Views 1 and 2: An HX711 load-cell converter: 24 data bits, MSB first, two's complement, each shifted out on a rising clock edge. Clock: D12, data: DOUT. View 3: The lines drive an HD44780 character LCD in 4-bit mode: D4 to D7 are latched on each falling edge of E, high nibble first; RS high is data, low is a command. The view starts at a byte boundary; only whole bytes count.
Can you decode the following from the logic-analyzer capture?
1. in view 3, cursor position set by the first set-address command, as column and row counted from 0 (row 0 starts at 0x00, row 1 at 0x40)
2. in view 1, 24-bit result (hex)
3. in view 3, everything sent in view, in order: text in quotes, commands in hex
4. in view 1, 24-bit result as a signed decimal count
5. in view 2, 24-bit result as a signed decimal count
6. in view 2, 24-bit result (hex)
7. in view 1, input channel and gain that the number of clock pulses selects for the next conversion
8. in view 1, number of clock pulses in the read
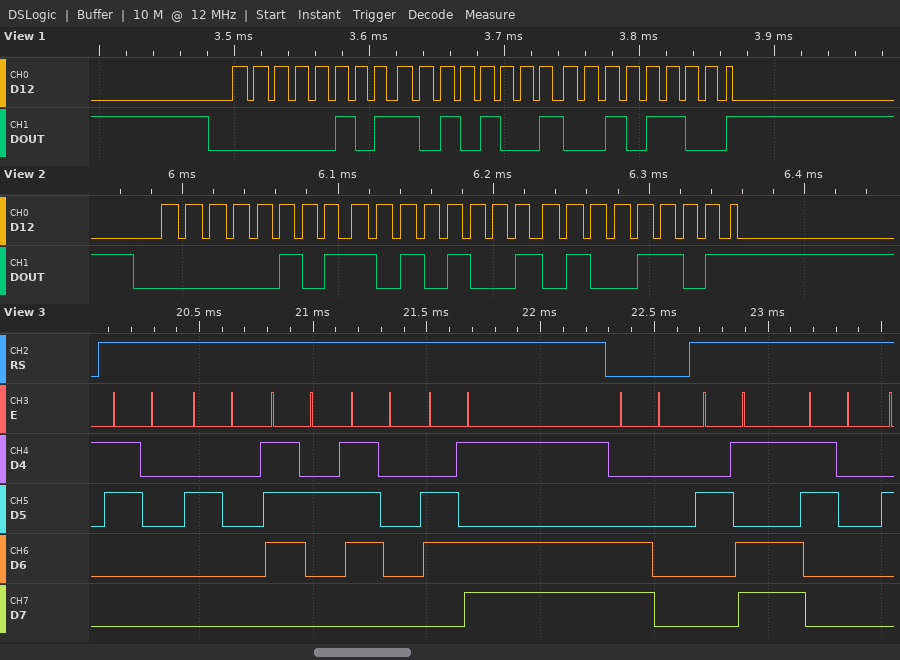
column 0, row 1
0x05A92C
"0 rpm" 0xC0 "-0"
370988
371021
0x05A94D
channel A, gain 128
25
